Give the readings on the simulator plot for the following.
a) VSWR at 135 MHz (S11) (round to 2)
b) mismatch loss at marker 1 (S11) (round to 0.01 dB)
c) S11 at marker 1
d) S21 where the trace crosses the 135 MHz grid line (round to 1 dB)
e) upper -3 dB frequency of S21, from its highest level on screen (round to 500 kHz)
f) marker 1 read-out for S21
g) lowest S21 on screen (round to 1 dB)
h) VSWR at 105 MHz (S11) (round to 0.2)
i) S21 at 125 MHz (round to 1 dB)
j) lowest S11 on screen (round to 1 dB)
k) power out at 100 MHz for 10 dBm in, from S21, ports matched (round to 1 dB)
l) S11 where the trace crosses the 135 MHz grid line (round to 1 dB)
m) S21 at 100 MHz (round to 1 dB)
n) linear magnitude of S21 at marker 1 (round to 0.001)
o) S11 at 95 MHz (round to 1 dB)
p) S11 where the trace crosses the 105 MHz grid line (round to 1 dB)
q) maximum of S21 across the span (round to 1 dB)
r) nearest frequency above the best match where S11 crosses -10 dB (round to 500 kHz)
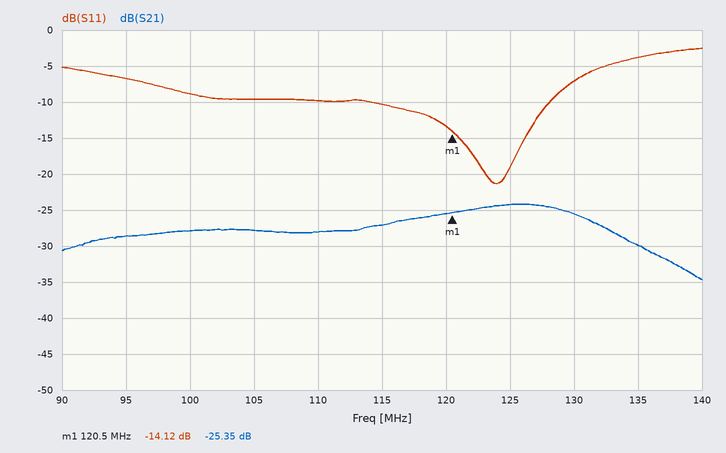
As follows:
4
0.17 dB
-14.12 dB
-30 dB
132.0 MHz
-25.35 dB
-35 dB
2.0
-24 dB
-21 dB
-18 dBm
-4 dB
-28 dB
0.054
-7 dB
-10 dB
-24 dB
128.0 MHz
